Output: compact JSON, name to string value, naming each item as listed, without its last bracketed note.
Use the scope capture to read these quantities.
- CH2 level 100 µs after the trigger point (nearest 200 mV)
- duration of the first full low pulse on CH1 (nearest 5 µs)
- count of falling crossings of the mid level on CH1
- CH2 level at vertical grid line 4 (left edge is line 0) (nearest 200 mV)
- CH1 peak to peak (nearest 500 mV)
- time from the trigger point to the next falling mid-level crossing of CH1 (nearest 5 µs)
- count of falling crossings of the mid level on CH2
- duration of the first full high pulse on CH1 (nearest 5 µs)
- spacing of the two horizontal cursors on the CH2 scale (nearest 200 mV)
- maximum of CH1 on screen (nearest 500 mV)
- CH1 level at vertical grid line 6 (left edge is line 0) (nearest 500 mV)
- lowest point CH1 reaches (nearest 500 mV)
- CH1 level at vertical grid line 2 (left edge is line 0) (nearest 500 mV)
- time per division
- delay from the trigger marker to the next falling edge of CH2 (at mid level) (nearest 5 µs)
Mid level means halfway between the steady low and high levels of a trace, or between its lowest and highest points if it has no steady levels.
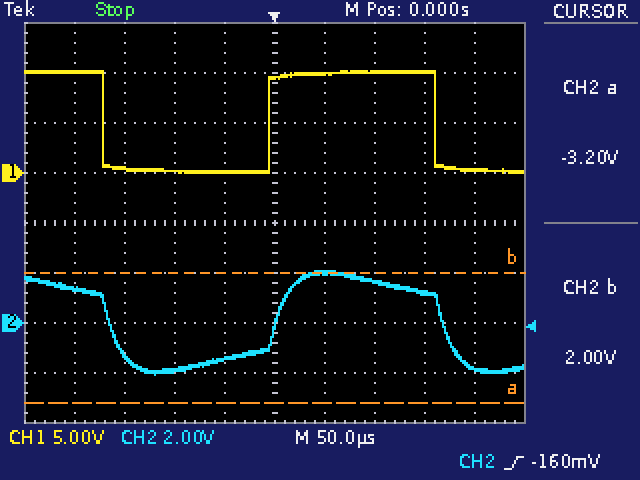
{"CH2 level 100 µs after the trigger point": "1.6 V", "duration of the first full low pulse on CH1": "165 µs", "count of falling crossings of the mid level on CH1": "2", "CH2 level at vertical grid line 4 (left edge is line 0)": "-1.4 V", "CH1 peak to peak": "10.0 V", "time from the trigger point to the next falling mid-level crossing of CH1": "160 µs", "count of falling crossings of the mid level on CH2": "2", "duration of the first full high pulse on CH1": "165 µs", "spacing of the two horizontal cursors on the CH2 scale": "5.2 V", "maximum of CH1 on screen": "10.0 V", "CH1 level at vertical grid line 6 (left edge is line 0)": "10.0 V", "lowest point CH1 reaches": "0.0 V", "CH1 level at vertical grid line 2 (left edge is line 0)": "500 mV", "time per division": "50 µs", "delay from the trigger marker to the next falling edge of CH2 (at mid level)": "170 µs"}
